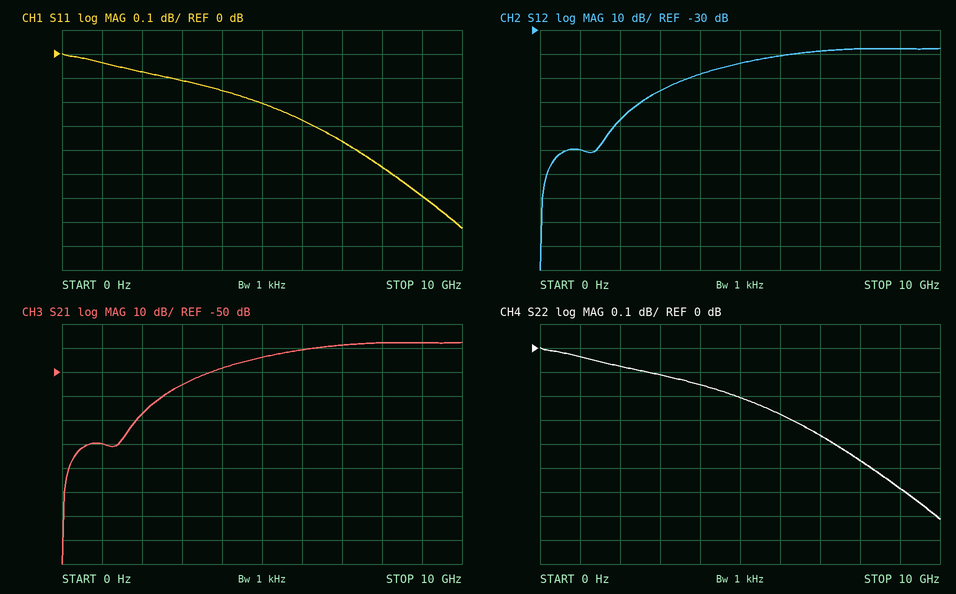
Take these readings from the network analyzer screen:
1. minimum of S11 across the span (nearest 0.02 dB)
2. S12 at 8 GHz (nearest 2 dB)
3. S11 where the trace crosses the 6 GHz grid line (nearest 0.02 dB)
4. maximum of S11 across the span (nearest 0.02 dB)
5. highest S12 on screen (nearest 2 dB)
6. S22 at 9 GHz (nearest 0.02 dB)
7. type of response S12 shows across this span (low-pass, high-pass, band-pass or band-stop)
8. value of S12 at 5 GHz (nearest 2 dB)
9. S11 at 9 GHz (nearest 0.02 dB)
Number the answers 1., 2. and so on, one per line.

1. -0.72 dB
2. -38 dB
3. -0.28 dB
4. 0.00 dB
5. -38 dB
6. -0.58 dB
7. high-pass
8. -44 dB
9. -0.60 dB
